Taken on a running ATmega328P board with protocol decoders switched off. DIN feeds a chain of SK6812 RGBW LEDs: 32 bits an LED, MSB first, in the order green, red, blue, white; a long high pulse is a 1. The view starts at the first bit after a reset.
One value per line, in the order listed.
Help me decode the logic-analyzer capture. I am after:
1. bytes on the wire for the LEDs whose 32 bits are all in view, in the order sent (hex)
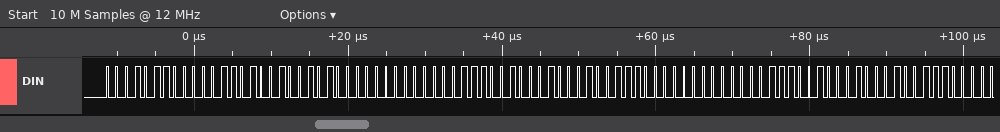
16 0D 25 00 07 22 27 00
